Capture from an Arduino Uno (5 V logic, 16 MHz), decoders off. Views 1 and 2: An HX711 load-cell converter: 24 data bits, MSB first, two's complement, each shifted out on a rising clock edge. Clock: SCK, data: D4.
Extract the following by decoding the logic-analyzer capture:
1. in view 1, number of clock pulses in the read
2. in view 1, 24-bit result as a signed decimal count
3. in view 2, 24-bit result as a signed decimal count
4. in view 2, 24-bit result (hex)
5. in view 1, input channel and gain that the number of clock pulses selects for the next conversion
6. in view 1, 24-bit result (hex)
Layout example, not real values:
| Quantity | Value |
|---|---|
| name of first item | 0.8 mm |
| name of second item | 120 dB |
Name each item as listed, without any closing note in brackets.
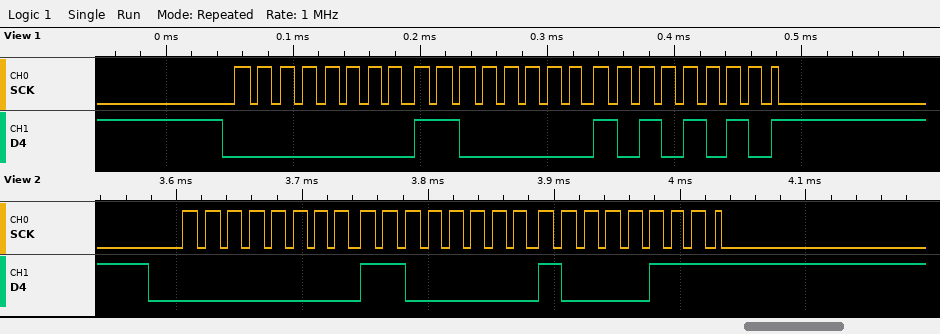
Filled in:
| Quantity | Value |
|---|---|
| in view 1, number of clock pulses in the read | 25 |
| in view 1, 24-bit result as a signed decimal count | 49322 |
| in view 2, 24-bit result as a signed decimal count | 49287 |
| in view 2, 24-bit result | 0x00C087 |
| in view 1, input channel and gain that the number of clock pulses selects for the next conversion | channel A, gain 128 |
| in view 1, 24-bit result | 0x00C0AA |
